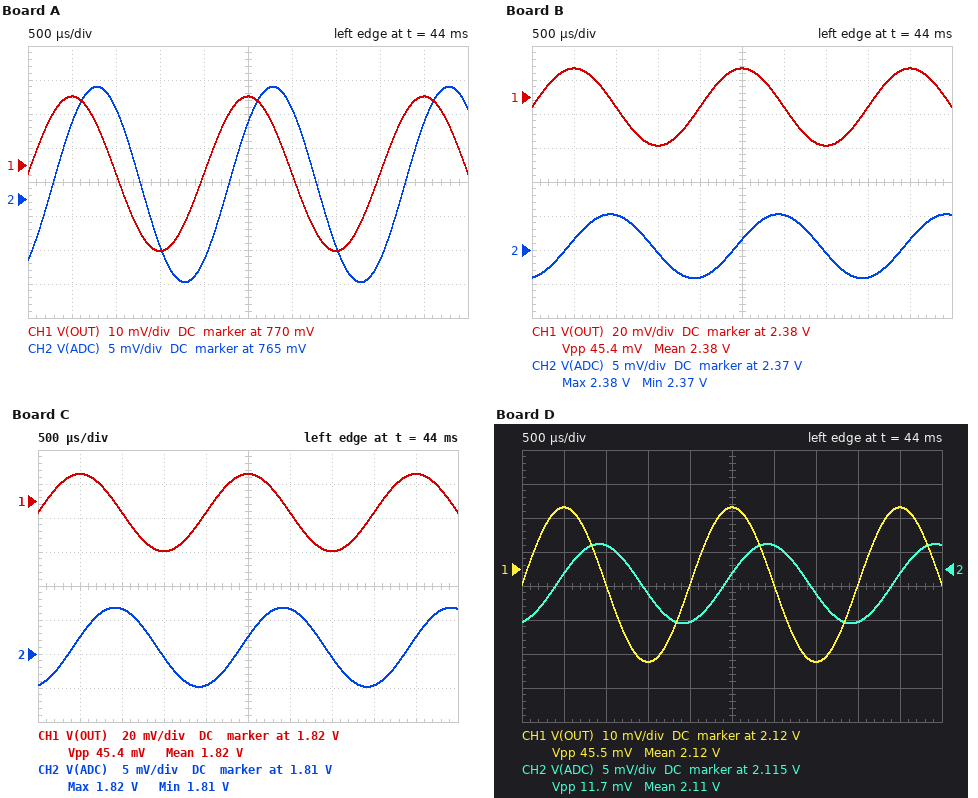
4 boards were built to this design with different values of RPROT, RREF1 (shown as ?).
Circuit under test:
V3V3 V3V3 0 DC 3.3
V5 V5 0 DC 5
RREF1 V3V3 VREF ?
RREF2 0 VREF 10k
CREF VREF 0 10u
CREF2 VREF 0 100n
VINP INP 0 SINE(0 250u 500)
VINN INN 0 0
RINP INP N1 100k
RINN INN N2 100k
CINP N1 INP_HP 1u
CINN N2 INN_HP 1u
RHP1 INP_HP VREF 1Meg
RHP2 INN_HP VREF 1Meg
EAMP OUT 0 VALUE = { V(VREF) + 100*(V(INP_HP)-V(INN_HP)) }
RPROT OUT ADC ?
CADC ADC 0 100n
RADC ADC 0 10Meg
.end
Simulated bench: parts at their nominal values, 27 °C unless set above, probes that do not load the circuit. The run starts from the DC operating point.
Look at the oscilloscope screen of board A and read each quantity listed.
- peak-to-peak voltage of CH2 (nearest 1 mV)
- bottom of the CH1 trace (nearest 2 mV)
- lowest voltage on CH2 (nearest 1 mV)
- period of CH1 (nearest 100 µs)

29 mV
744 mV
753 mV
2.0 ms
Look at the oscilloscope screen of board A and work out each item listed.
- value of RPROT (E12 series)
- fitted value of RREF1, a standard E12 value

3.9 kΩ
33 kΩ
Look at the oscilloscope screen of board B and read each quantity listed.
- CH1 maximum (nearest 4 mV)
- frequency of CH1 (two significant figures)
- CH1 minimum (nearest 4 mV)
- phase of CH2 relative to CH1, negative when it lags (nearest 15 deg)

2.396 V
500 Hz
2.352 V
-75 deg
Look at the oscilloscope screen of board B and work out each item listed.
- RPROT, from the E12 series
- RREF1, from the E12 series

15 kΩ
3.9 kΩ
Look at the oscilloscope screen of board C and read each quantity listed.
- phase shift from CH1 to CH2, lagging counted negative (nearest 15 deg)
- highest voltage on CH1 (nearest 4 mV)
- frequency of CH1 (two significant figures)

-75 deg
1.836 V
500 Hz
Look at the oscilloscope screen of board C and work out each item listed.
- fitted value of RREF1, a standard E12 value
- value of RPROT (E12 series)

8.2 kΩ
12 kΩ
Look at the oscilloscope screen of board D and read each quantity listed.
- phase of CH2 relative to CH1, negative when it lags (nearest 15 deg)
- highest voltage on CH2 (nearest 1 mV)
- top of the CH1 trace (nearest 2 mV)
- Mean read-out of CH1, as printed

-75 deg
2.119 V
2.138 V
2.12 V
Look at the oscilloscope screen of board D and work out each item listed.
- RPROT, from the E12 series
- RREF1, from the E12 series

12 kΩ
5.6 kΩ
